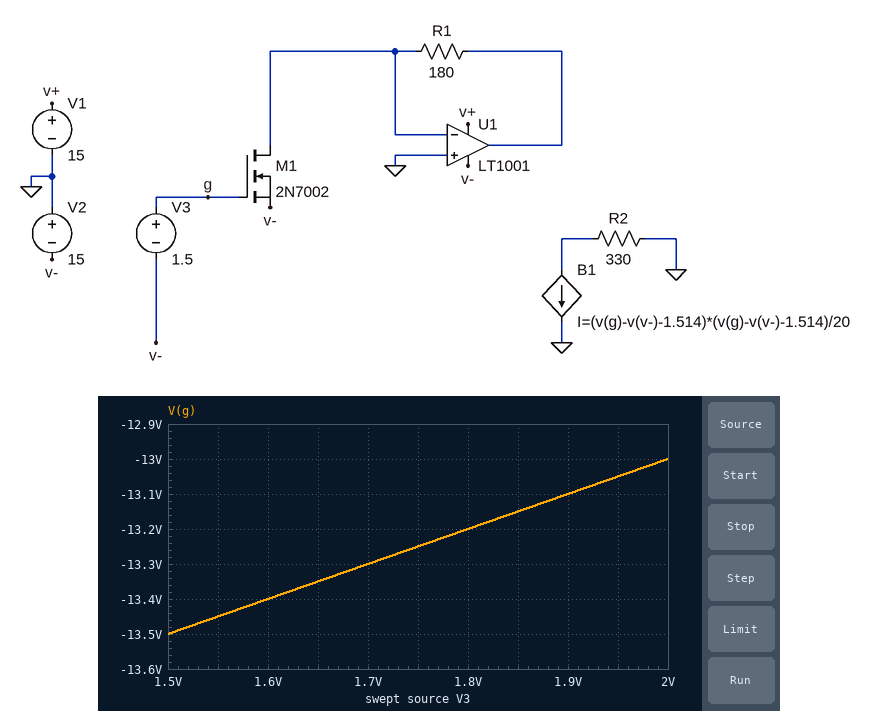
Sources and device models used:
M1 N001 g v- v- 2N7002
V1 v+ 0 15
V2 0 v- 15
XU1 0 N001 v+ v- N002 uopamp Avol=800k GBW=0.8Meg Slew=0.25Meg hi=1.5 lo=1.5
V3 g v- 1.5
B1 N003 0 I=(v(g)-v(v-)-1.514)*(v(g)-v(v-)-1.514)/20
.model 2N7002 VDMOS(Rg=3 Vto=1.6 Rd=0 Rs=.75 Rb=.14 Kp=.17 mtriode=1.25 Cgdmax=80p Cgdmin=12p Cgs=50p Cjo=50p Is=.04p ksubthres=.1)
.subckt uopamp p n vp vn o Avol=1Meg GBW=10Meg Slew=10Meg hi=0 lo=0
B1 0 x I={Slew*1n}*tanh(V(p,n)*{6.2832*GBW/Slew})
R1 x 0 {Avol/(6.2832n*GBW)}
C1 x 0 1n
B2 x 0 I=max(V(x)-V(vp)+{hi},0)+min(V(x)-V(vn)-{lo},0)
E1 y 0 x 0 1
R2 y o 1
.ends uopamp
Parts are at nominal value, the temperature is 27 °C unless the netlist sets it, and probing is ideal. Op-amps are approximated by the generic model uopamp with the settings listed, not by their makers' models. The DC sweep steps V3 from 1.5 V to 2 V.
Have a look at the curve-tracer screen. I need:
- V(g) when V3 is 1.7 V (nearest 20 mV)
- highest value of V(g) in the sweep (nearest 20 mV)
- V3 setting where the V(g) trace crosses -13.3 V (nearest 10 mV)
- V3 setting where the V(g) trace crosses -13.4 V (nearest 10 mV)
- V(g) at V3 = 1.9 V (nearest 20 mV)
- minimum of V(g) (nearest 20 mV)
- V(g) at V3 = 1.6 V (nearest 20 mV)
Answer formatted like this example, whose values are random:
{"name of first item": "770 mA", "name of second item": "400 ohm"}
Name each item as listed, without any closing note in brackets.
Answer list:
{"V(g) when V3 is 1.7 V": "-13.30 V", "highest value of V(g) in the sweep": "-13.00 V", "V3 setting where the V(g) trace crosses -13.3 V": "1.70 V", "V3 setting where the V(g) trace crosses -13.4 V": "1.60 V", "V(g) at V3 = 1.9 V": "-13.10 V", "minimum of V(g)": "-13.50 V", "V(g) at V3 = 1.6 V": "-13.40 V"}
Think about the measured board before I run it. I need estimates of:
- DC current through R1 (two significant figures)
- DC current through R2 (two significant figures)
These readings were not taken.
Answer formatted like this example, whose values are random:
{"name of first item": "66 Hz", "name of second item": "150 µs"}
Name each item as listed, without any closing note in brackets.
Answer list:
{"DC current through R1": "83 µA", "DC current through R2": "9.8 µA"}
